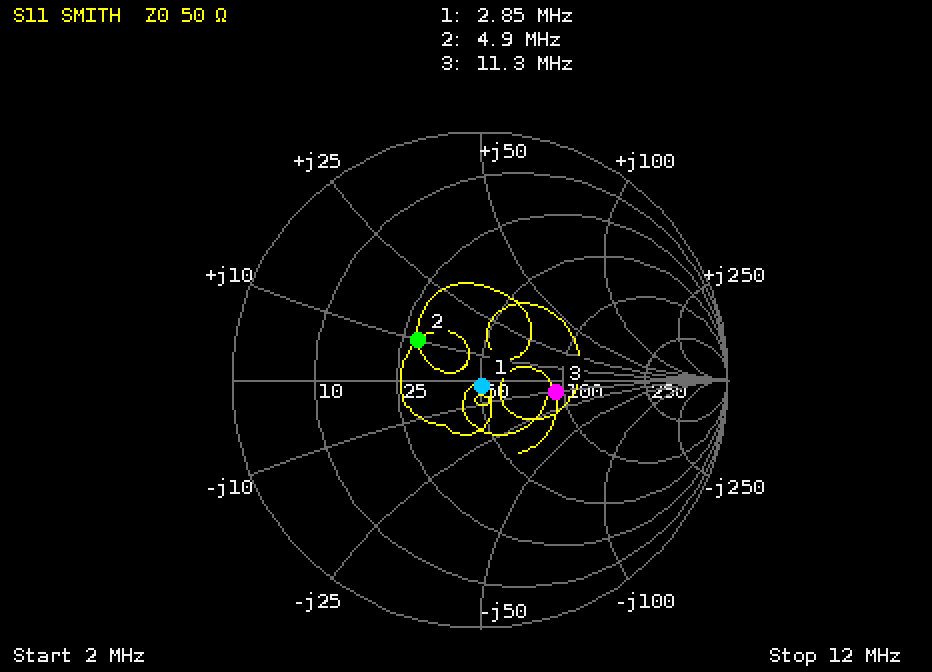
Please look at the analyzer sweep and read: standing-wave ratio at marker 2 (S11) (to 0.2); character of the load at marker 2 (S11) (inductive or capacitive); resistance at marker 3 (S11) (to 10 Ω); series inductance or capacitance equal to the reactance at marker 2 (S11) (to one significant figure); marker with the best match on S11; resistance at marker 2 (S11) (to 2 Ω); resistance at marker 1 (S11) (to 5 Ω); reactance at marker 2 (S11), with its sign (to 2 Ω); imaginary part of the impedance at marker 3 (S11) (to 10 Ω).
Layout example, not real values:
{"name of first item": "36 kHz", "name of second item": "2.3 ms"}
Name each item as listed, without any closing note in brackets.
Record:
{"standing-wave ratio at marker 2 (S11)": "1.8", "character of the load at marker 2 (S11)": "inductive", "resistance at marker 3 (S11)": "90 Ω", "series inductance or capacitance equal to the reactance at marker 2 (S11)": "300 nH", "marker with the best match on S11": "marker 1", "resistance at marker 2 (S11)": "28 Ω", "resistance at marker 1 (S11)": "50 Ω", "reactance at marker 2 (S11), with its sign": "+10 Ω", "imaginary part of the impedance at marker 3 (S11)": "-10 Ω"}
